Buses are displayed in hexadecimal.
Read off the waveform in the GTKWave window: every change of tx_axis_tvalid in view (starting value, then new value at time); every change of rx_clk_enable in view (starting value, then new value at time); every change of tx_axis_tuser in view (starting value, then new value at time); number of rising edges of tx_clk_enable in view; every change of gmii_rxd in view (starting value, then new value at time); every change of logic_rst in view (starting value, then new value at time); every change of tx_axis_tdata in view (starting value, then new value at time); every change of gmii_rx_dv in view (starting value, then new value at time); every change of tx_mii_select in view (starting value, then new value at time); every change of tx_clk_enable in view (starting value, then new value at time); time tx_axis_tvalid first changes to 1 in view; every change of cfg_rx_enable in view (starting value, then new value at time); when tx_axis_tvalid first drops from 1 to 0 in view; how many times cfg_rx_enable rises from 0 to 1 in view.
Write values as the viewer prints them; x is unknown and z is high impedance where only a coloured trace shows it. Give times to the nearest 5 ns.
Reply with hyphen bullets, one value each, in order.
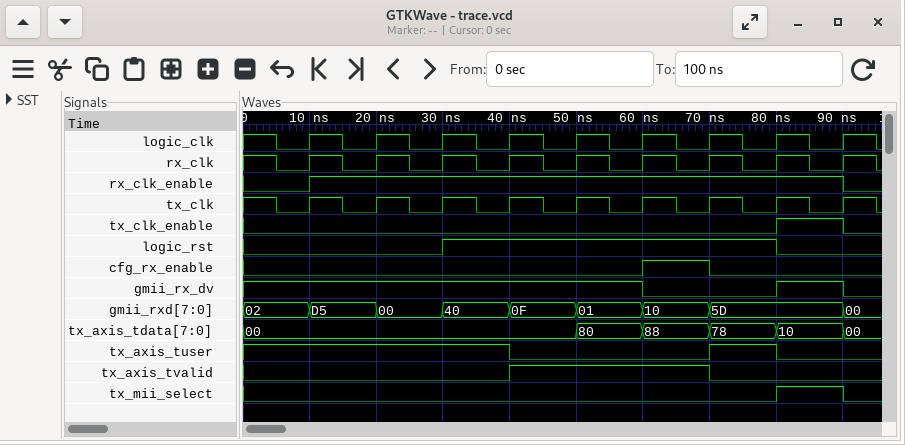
- 0, 1 at 40 ns, 0 at 70 ns
- 0, 1 at 10 ns, 0 at 90 ns
- 1, 0 at 40 ns, 1 at 70 ns, 0 at 80 ns
- 1
- 02, D5 at 10 ns, 00 at 20 ns, 40 at 30 ns, 0F at 40 ns, 01 at 50 ns, 10 at 60 ns, 5D at 70 ns, 00 at 90 ns
- 0, 1 at 30 ns, 0 at 80 ns
- 00, 80 at 50 ns, 88 at 60 ns, 78 at 70 ns, 10 at 80 ns, 00 at 90 ns
- 1, 0 at 60 ns, 1 at 80 ns, 0 at 90 ns
- 0, 1 at 80 ns, 0 at 90 ns
- 0, 1 at 80 ns, 0 at 90 ns
- 40 ns
- 0, 1 at 60 ns, 0 at 70 ns
- 70 ns
- 1
